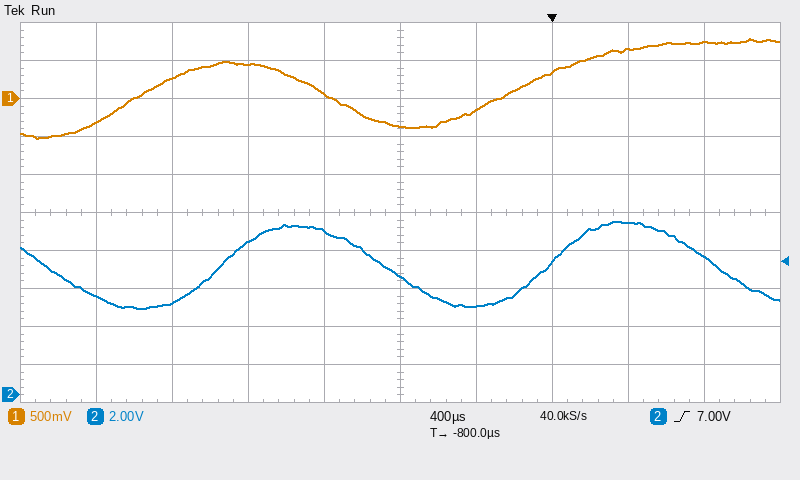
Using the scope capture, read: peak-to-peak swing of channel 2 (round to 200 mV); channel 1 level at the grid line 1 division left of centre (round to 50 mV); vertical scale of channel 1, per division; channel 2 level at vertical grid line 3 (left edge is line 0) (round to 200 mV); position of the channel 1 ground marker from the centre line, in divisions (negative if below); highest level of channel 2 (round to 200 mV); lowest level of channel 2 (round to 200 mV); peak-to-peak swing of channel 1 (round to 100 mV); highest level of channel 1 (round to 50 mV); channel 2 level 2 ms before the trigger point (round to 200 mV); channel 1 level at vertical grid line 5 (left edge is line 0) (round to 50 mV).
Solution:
4.6 V
50 mV
500 mV
8.0 V
+3.0 div
9.2 V
4.6 V
1.30 V
800 mV
4.8 V
-350 mV
